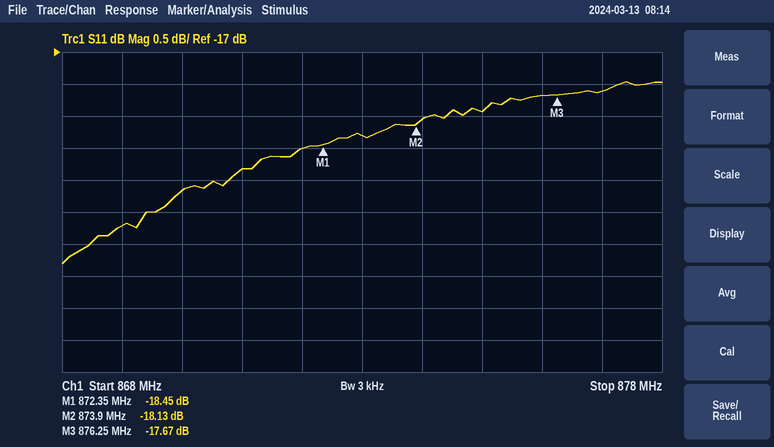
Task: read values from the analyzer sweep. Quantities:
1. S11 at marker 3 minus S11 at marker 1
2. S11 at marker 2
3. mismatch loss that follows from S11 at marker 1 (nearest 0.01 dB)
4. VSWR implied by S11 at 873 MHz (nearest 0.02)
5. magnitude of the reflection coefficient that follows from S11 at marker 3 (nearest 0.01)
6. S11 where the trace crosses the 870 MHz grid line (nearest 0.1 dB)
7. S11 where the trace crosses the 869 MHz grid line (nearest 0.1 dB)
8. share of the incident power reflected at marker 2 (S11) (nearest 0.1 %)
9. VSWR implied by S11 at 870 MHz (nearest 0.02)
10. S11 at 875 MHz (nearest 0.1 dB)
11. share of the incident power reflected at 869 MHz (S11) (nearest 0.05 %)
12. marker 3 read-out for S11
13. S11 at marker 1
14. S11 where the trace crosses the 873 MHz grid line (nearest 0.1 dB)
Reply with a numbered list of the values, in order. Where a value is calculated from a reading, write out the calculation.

1. -17.67 − (-18.45) = 0.78 dB
2. -18.13 dB
3. −10 log10(1 − 10^(-18.45/10)) ≈ 0.06 dB
4. |Γ| = 10^(-18.3/20) = 0.1216; VSWR = (1 + 0.1216)/(1 − 0.1216) ≈ 1.28
5. 10^(-17.67/20) ≈ 0.13
6. -19.2 dB
7. -19.7 dB
8. 10^(-18.13/10) ≈ 1.5 %
9. |Γ| = 10^(-19.2/20) = 0.1096; VSWR = (1 + 0.1096)/(1 − 0.1096) ≈ 1.25, so 1.24 to the nearest 0.02
10. -17.9 dB
11. 10^(-19.7/10) ≈ 1.07 %, so 1.05 % to the nearest 0.05 %
12. -17.67 dB
13. -18.45 dB
14. -18.3 dB
